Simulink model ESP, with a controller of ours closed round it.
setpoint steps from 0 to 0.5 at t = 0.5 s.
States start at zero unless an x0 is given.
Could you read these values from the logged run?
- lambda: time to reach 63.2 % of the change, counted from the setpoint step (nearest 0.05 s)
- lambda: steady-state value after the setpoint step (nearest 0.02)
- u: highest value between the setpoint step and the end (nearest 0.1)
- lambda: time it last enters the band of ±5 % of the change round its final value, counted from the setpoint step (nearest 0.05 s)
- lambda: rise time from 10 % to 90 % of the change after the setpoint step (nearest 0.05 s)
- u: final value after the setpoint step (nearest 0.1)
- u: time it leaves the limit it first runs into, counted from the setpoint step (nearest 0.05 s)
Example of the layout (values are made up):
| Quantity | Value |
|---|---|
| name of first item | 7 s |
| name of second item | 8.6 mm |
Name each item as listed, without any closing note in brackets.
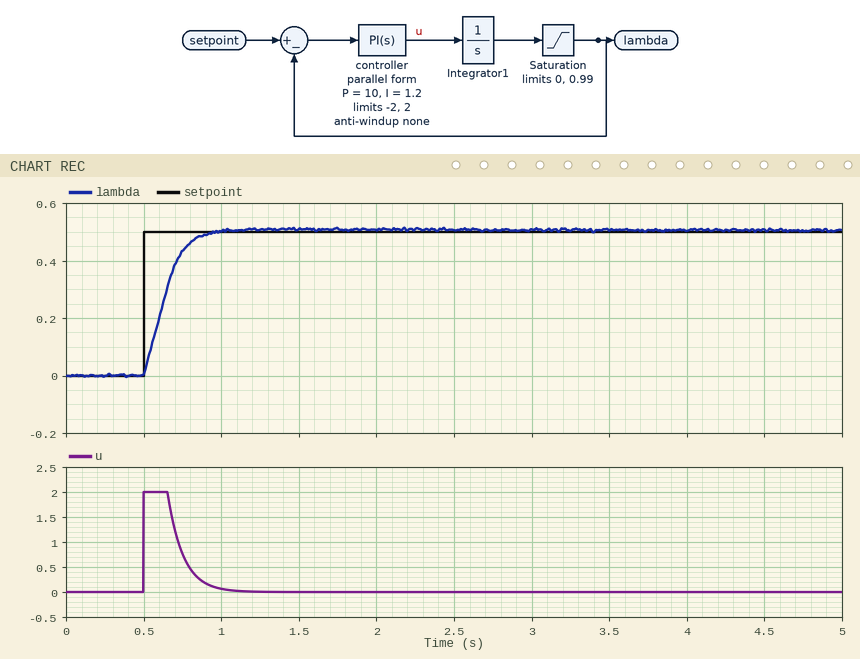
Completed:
| Quantity | Value |
|---|---|
| lambda: time to reach 63.2 % of the change, counted from the setpoint step | 0.15 s |
| lambda: steady-state value after the setpoint step | 0.50 |
| u: highest value between the setpoint step and the end | 2.0 |
| lambda: time it last enters the band of ±5 % of the change round its final value, counted from the setpoint step | 0.35 s |
| lambda: rise time from 10 % to 90 % of the change after the setpoint step | 0.25 s |
| u: final value after the setpoint step | 0.0 |
| u: time it leaves the limit it first runs into, counted from the setpoint step | 0.15 s |
